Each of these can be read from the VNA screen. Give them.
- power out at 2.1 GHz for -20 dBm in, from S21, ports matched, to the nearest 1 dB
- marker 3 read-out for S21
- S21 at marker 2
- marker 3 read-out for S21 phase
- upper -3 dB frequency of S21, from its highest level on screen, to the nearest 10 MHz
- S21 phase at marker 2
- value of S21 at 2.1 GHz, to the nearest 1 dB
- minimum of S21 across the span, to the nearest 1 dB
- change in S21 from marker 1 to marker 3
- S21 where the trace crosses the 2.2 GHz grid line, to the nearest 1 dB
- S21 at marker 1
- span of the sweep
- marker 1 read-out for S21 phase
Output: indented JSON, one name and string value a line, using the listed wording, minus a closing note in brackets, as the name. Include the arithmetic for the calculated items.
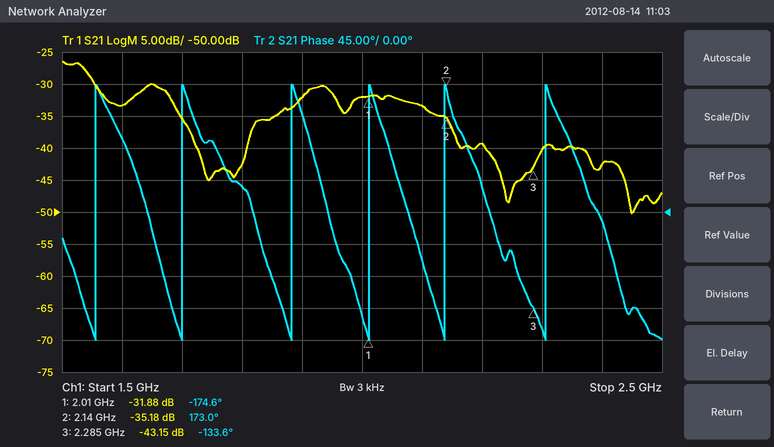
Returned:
{
  "power out at 2.1 GHz for -20 dBm in, from S21, ports matched, to the nearest 1 dB": "-20 dBm + (-33 dB) = -53 dBm",
  "marker 3 read-out for S21": "-43.15 dB",
  "S21 at marker 2": "-35.18 dB",
  "marker 3 read-out for S21 phase": "-133.6°",
  "upper -3 dB frequency of S21, from its highest level on screen, to the nearest 10 MHz": "1.55 GHz",
  "S21 phase at marker 2": "173.0°",
  "value of S21 at 2.1 GHz, to the nearest 1 dB": "-33 dB",
  "minimum of S21 across the span, to the nearest 1 dB": "-50 dB",
  "change in S21 from marker 1 to marker 3": "-43.15 − (-31.88) = -11.27 dB",
  "S21 where the trace crosses the 2.2 GHz grid line, to the nearest 1 dB": "-39 dB",
  "S21 at marker 1": "-31.88 dB",
  "span of the sweep": "1 GHz",
  "marker 1 read-out for S21 phase": "-174.6°"
}
